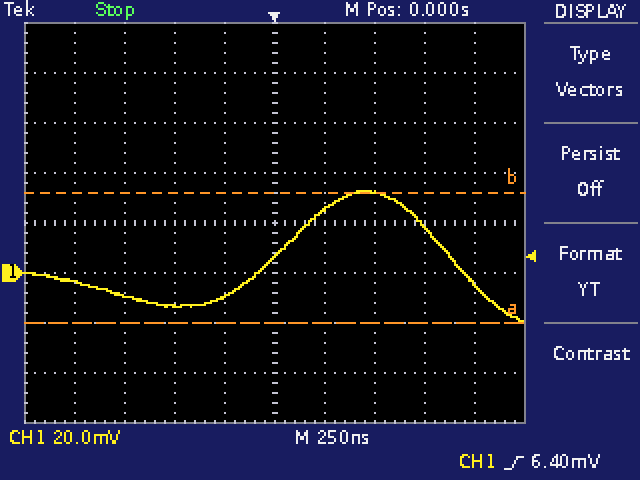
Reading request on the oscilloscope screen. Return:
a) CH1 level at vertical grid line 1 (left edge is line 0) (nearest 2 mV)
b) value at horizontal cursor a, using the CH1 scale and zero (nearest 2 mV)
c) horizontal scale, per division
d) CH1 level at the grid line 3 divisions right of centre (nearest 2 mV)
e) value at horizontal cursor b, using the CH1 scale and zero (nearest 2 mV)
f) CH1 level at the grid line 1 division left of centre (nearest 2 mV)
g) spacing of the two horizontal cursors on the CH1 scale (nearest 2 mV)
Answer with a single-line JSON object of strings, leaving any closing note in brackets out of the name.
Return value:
{"CH1 level at vertical grid line 1 (left edge is line 0)": "-4 mV", "value at horizontal cursor a, using the CH1 scale and zero": "-20 mV", "horizontal scale, per division": "250 ns", "CH1 level at the grid line 3 divisions right of centre": "18 mV", "value at horizontal cursor b, using the CH1 scale and zero": "32 mV", "CH1 level at the grid line 1 division left of centre": "-10 mV", "spacing of the two horizontal cursors on the CH1 scale": "52 mV"}
